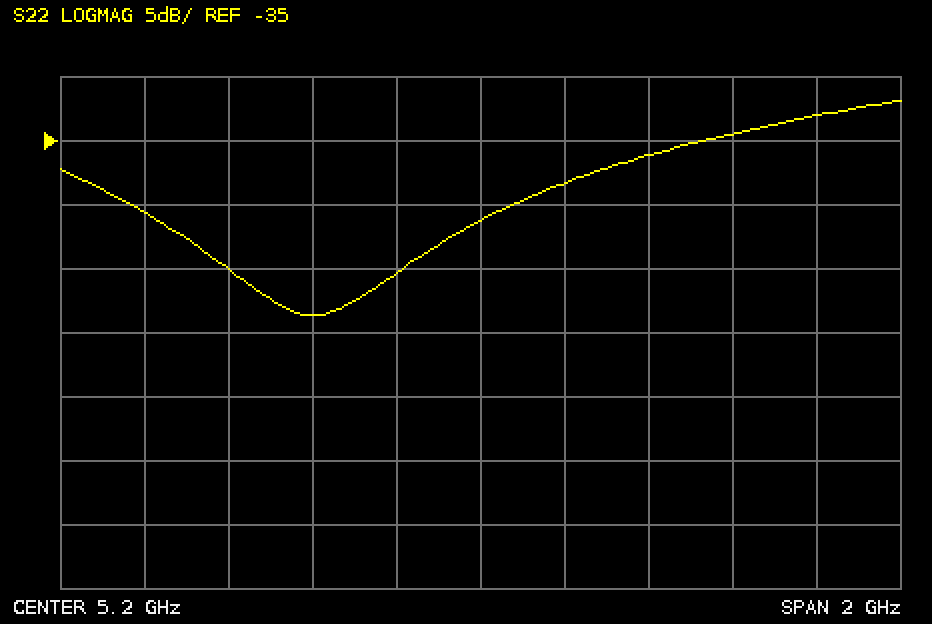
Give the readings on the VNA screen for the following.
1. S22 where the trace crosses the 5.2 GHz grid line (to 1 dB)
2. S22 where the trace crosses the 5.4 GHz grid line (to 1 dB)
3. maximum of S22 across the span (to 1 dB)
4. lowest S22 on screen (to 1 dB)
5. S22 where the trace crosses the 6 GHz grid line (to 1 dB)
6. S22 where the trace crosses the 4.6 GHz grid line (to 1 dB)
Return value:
-41 dB
-38 dB
-32 dB
-49 dB
-33 dB
-45 dB
